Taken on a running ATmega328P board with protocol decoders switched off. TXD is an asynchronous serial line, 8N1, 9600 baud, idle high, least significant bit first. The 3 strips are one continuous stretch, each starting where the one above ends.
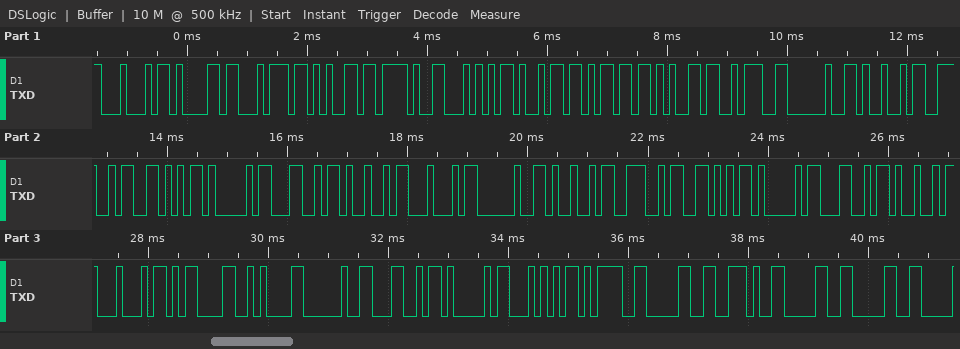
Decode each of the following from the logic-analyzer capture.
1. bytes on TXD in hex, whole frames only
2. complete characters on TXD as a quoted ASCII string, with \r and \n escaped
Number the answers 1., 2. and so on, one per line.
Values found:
1. 0x44 0x61 0x74 0x65 0x2F 0x54 0x69 0x6D 0x65 0x3A 0x20 0x49 0x4E 0x56 0x41 0x4C 0x49 0x44 0x20 0x49 0x4E 0x56 0x41 0x4C 0x49 0x44 0x0D 0x0A 0x20 0x4C 0x41 0x54 0x3D 0x30 0x2E 0x30 0x30
2. "Date/Time: INVALID INVALID\r\n LAT=0.00"
